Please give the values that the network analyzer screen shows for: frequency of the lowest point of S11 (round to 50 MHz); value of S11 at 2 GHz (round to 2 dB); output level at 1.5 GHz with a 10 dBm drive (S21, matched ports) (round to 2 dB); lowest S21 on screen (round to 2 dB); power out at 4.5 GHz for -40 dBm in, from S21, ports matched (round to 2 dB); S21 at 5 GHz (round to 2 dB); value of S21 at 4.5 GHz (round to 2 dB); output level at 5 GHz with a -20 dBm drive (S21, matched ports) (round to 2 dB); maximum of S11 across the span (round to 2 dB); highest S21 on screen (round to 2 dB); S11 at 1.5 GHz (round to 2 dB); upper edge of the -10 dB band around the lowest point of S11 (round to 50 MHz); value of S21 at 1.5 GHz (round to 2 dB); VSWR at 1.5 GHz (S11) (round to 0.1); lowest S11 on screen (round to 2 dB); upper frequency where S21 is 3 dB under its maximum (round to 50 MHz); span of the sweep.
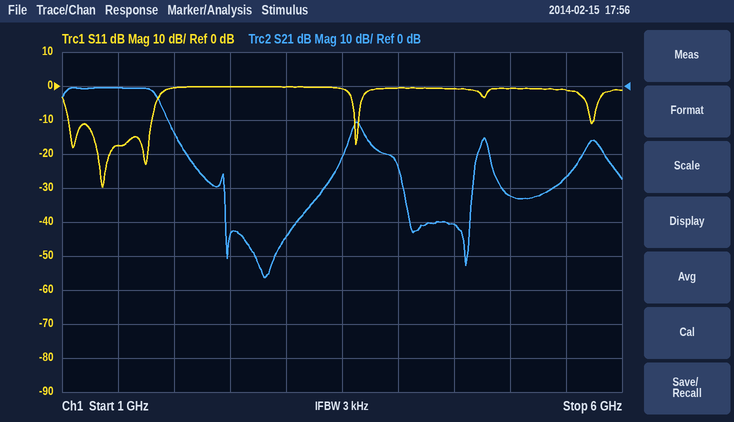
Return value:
1.35 GHz
0 dB
10 dBm
-56 dB
-80 dBm
-32 dB
-40 dB
-52 dBm
0 dB
0 dB
-18 dB
1.80 GHz
0 dB
1.3
-30 dB
1.85 GHz
5 GHz
